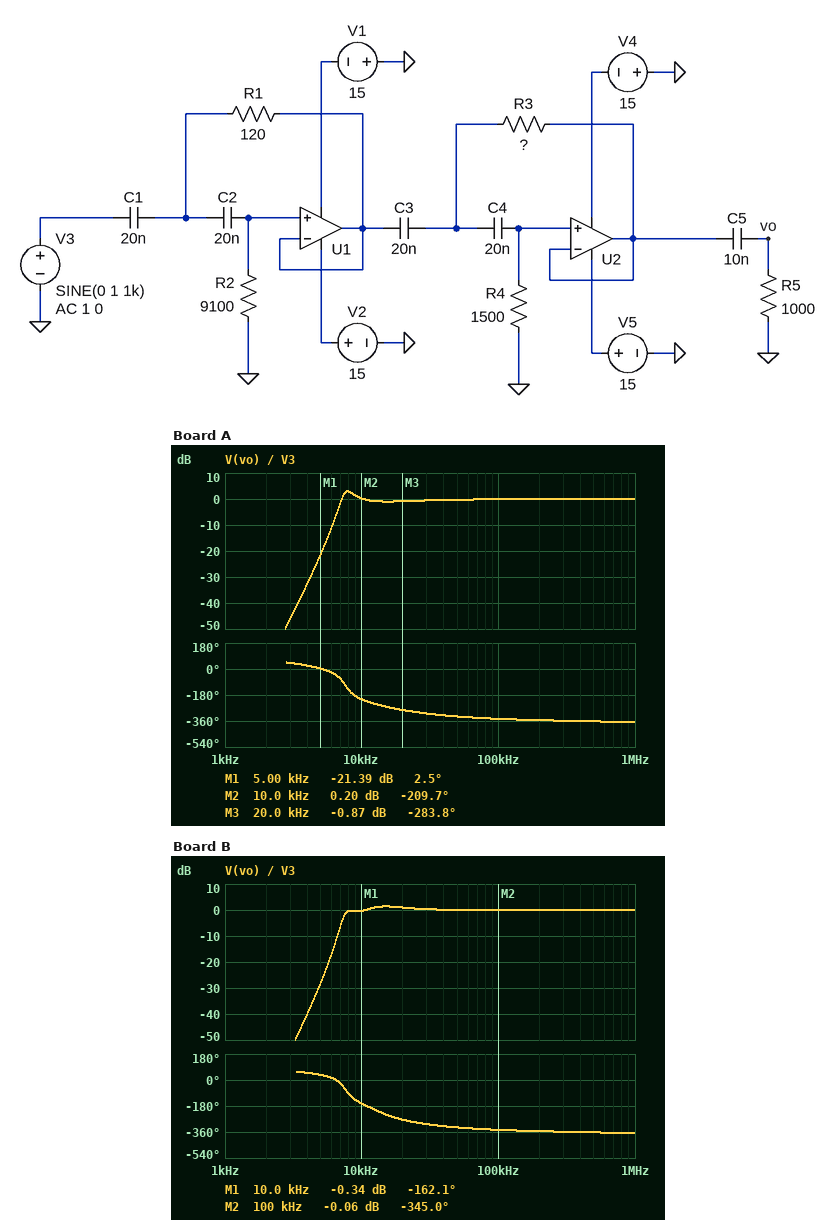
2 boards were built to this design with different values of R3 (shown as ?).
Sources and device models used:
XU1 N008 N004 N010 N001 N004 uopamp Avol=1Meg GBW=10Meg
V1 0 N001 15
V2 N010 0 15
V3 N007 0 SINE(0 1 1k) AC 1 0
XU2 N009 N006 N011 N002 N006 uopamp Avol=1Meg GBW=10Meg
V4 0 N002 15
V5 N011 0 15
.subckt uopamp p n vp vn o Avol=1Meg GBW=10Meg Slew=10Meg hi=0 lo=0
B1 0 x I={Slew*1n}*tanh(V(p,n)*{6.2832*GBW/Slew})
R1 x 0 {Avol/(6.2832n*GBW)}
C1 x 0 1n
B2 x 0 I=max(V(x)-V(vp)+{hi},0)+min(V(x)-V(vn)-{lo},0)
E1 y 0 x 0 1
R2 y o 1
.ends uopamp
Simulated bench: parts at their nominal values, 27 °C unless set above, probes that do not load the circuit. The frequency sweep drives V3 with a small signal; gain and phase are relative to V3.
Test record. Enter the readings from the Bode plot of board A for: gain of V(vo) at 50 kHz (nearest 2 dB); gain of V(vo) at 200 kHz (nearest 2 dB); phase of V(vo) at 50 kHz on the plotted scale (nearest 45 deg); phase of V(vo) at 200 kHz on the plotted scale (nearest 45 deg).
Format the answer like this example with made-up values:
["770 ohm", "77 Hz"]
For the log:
["0 dB", "0 dB", "-315 deg", "-360 deg"]
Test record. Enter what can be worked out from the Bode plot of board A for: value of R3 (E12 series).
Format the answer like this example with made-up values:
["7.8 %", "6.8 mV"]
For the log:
["680 Ω"]
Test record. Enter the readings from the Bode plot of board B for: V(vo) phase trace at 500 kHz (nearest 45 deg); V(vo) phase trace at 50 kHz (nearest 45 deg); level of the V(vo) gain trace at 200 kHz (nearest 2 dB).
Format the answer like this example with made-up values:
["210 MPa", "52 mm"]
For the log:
["-360 deg", "-315 deg", "0 dB"]
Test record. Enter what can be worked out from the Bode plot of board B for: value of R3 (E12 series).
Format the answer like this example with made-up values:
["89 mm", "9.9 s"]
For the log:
["270 Ω"]
